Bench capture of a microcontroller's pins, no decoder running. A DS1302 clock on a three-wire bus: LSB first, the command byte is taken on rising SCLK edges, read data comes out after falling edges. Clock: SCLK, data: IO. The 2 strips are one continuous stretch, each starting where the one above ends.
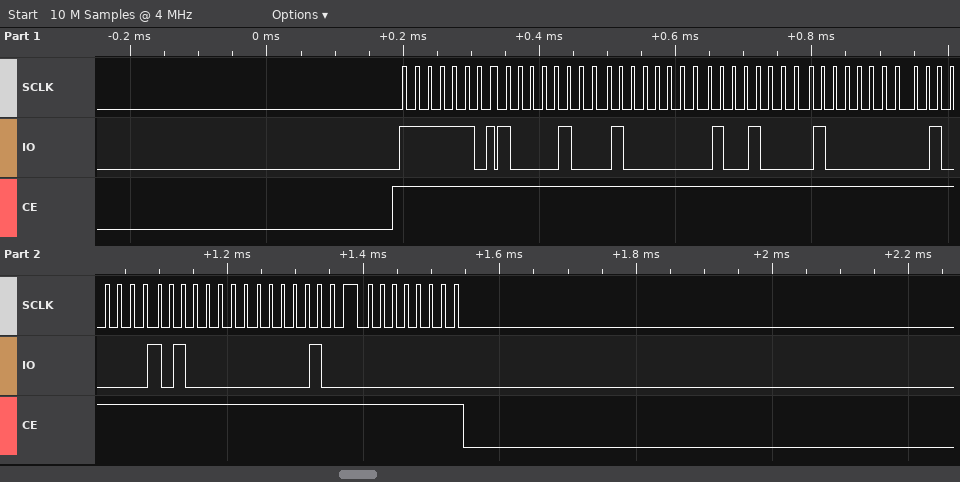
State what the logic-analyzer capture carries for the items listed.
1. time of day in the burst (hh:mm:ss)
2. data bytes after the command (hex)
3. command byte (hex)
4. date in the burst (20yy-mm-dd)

12:02:21
21 02 12 02 04 05 20 00
0xBF
2020-04-02
